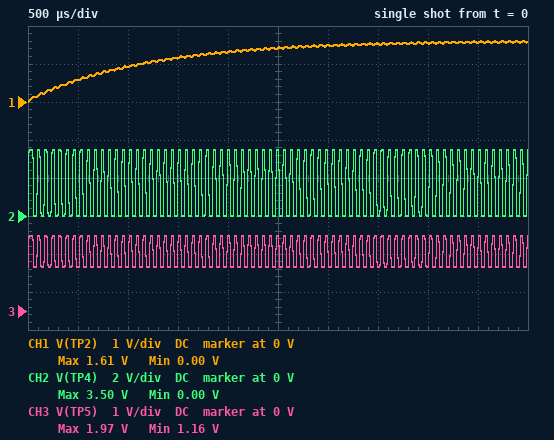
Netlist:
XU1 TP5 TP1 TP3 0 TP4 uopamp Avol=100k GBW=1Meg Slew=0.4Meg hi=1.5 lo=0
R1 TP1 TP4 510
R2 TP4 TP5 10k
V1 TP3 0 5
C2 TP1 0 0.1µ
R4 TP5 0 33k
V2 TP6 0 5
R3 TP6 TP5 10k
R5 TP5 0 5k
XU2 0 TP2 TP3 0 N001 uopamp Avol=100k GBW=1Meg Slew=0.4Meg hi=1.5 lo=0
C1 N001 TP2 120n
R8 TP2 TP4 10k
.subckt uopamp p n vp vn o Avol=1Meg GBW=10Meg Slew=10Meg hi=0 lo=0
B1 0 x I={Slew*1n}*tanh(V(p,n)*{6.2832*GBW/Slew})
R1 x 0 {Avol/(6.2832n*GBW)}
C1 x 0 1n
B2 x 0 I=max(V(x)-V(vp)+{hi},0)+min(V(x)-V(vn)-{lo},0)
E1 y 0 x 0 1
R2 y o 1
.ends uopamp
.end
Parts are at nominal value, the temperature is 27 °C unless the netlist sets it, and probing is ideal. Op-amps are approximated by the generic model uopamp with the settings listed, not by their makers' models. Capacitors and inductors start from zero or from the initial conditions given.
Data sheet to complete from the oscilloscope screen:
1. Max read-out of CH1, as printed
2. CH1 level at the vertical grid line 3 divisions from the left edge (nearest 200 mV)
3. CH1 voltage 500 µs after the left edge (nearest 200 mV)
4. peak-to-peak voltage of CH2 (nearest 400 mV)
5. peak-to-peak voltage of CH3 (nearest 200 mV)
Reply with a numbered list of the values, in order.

1. 1.61 V
2. 1.2 V
3. 600 mV
4. 3.6 V
5. 800 mV
